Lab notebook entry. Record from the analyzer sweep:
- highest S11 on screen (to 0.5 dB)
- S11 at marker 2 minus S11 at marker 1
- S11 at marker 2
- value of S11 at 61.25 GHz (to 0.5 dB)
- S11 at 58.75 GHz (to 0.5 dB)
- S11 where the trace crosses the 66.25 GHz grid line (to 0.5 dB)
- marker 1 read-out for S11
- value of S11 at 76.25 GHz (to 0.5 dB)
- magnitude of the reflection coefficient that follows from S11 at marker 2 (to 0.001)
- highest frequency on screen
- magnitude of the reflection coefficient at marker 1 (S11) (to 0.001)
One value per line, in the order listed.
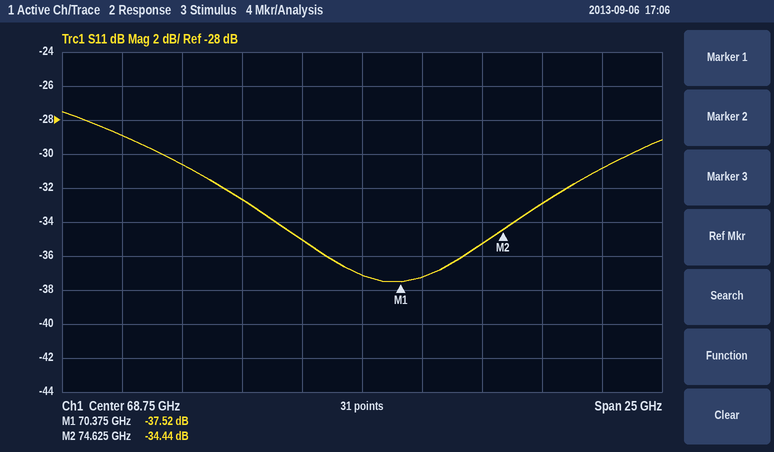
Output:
-27.5 dB
3.08 dB
-34.44 dB
-30.5 dB
-29.0 dB
-35.0 dB
-37.52 dB
-33.0 dB
0.019
81.25 GHz
0.013
